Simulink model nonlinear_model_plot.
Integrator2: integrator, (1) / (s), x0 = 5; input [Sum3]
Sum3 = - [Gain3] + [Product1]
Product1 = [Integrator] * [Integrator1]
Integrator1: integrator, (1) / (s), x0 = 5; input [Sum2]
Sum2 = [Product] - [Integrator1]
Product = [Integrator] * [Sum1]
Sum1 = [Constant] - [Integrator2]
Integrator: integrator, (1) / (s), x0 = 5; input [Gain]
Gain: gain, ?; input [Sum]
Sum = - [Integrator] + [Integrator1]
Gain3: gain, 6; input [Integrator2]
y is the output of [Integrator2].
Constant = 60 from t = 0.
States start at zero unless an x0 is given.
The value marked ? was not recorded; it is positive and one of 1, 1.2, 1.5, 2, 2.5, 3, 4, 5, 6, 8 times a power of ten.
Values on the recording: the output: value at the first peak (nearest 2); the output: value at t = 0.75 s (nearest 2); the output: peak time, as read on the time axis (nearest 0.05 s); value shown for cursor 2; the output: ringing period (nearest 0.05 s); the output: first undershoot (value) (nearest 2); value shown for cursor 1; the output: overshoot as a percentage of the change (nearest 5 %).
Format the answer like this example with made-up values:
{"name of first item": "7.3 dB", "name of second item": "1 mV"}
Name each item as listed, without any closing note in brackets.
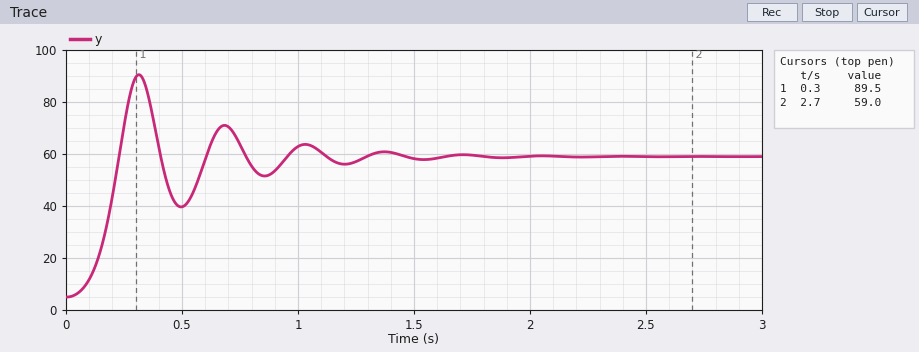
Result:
{"the output: value at the first peak": "90", "the output: value at t = 0.75 s": "64", "the output: peak time, as read on the time axis": "0.30 s", "value shown for cursor 2": "59.0", "the output: ringing period": "0.35 s", "the output: first undershoot (value)": "40", "value shown for cursor 1": "89.5", "the output: overshoot as a percentage of the change": "60 %"}
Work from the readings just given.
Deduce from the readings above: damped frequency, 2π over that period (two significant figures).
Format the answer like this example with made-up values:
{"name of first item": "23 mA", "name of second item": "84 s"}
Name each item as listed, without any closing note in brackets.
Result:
{"damped frequency, 2π over that period": "18 rad/s"}
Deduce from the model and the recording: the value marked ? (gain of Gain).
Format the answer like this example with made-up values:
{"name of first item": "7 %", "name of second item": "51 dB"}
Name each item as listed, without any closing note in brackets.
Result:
{"the value marked ?": "1.5"}
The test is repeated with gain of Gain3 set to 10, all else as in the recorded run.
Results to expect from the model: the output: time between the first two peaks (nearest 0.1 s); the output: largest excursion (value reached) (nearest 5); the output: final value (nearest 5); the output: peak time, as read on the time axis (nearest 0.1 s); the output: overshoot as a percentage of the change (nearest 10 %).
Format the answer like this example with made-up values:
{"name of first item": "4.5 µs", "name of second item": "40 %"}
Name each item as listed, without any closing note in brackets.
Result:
{"the output: time between the first two peaks": "0.3 s", "the output: largest excursion (value reached)": "85", "the output: final value": "60", "the output: peak time, as read on the time axis": "0.3 s", "the output: overshoot as a percentage of the change": "50 %"}
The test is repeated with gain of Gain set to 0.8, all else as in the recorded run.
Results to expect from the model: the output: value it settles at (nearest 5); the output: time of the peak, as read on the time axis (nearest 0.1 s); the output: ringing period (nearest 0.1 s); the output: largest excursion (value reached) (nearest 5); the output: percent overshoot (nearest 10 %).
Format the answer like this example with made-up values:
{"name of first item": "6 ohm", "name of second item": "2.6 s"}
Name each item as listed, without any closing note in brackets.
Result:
{"the output: value it settles at": "60", "the output: time of the peak, as read on the time axis": "0.4 s", "the output: ringing period": "0.4 s", "the output: largest excursion (value reached)": "85", "the output: percent overshoot": "50 %"}
